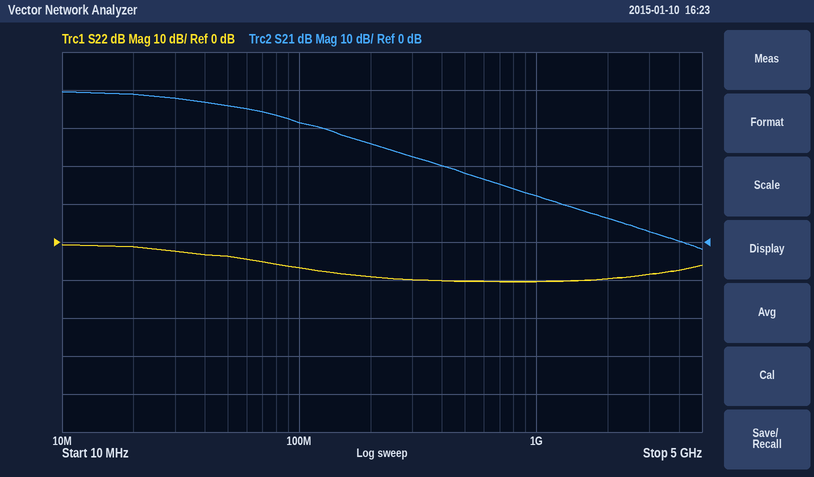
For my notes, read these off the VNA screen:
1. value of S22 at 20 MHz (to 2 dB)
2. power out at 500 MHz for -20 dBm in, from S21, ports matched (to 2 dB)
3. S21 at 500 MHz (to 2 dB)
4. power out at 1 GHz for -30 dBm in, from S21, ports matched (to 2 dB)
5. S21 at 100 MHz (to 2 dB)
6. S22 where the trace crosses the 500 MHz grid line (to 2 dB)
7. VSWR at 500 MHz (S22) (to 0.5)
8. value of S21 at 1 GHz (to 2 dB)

-2 dB
-2 dBm
18 dB
-18 dBm
32 dB
-10 dB
2.0
12 dB
